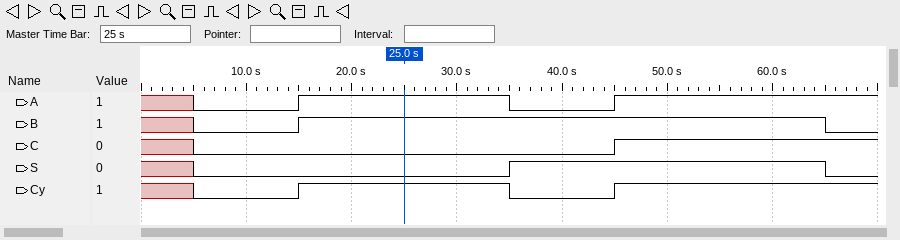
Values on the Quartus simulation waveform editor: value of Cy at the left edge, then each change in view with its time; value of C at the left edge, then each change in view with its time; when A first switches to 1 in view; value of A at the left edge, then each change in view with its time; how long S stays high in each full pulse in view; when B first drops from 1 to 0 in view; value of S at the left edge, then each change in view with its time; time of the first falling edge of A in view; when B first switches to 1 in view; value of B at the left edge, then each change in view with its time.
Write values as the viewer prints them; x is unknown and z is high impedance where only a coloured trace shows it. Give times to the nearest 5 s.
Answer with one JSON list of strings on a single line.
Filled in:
["x, 0 at 5 s, 1 at 15 s, 0 at 35 s, 1 at 45 s", "x, 0 at 5 s, 1 at 45 s", "15 s", "x, 0 at 5 s, 1 at 15 s, 0 at 35 s, 1 at 45 s", "30 s", "65 s", "x, 0 at 5 s, 1 at 35 s, 0 at 65 s", "35 s", "15 s", "x, 0 at 5 s, 1 at 15 s, 0 at 65 s"]
